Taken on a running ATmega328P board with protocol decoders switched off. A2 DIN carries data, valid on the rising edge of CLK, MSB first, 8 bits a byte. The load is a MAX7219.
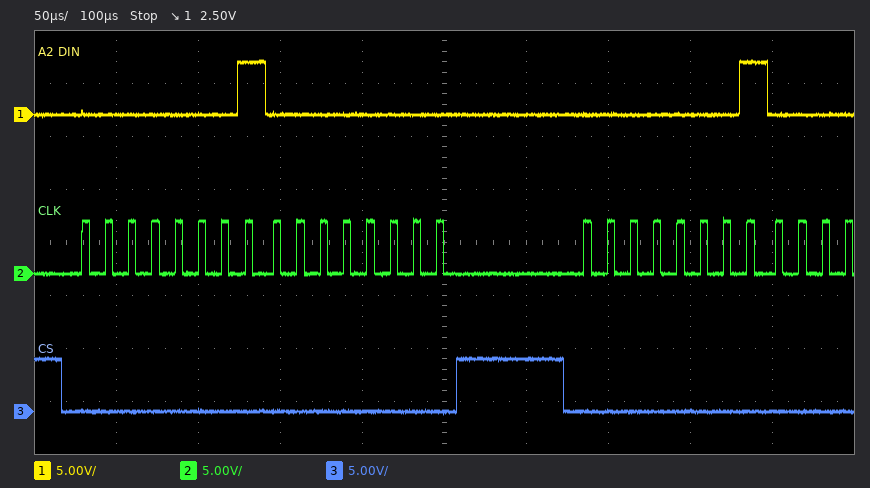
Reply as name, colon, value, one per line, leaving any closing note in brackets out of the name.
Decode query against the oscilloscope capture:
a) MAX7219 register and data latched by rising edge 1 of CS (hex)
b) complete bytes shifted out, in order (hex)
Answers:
MAX7219 register and data latched by rising edge 1 of CS: register 0x1, data 0x00
complete bytes shifted out, in order: 01 00 01
